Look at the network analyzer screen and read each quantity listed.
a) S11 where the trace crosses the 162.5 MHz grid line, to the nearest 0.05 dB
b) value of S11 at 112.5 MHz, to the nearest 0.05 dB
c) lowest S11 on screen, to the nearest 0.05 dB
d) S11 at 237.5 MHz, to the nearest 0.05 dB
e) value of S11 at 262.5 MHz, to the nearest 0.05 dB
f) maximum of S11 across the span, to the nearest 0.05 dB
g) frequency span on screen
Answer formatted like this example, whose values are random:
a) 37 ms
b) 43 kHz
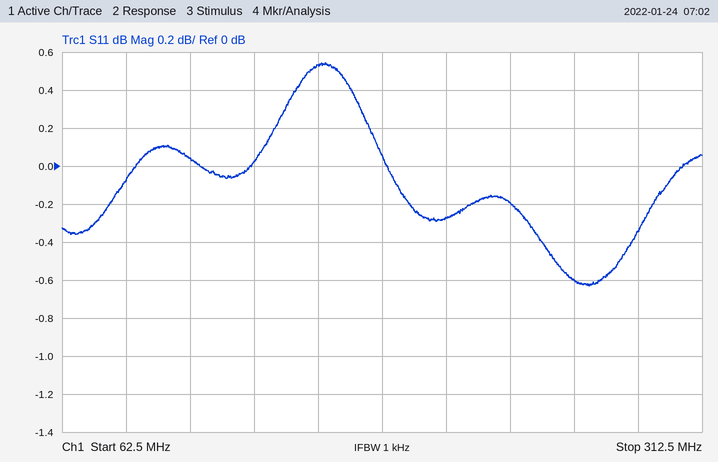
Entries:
a) 0.55 dB
b) 0.05 dB
c) -0.65 dB
d) -0.20 dB
e) -0.60 dB
f) 0.55 dB
g) 250 MHz
